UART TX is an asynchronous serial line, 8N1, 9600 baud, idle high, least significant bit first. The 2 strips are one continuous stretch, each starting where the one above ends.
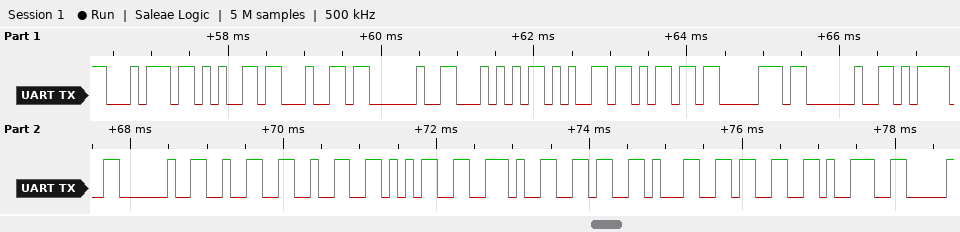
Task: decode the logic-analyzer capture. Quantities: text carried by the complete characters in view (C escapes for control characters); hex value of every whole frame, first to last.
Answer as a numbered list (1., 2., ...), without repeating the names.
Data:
1. "ted Temp = 225.6139"
2. 74 65 64 20 54 65 6D 70 20 3D 20 32 32 35 2E 36 31 33 39
